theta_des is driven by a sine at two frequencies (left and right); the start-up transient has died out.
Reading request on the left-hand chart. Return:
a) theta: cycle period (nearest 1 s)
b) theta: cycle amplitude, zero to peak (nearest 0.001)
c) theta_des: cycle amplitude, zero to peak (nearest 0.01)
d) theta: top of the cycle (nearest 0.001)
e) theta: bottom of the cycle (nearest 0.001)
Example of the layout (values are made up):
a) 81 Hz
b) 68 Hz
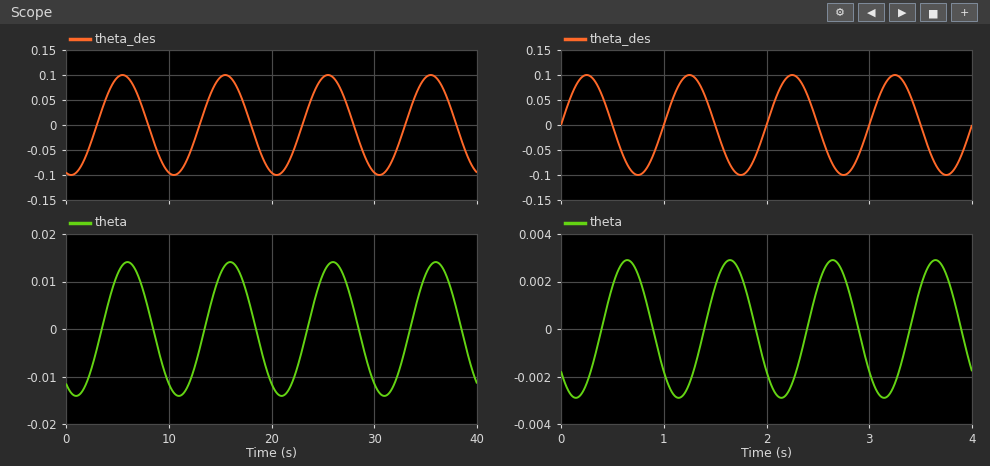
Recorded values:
a) 10 s
b) 0.014
c) 0.10
d) 0.014
e) -0.014
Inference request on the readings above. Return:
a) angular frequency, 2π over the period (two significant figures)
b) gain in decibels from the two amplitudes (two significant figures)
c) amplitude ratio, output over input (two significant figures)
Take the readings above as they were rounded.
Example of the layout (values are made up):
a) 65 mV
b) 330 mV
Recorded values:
a) 0.63 rad/s
b) -17 dB
c) 0.14
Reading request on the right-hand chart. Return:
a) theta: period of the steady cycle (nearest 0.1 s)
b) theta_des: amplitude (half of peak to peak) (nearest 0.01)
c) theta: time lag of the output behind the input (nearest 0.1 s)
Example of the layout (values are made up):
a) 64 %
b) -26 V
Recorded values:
a) 1.0 s
b) 0.10
c) 0.4 s
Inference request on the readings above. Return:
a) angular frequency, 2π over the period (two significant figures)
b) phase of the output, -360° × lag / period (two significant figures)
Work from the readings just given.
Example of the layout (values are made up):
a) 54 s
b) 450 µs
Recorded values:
a) 6.3 rad/s
b) -140°
